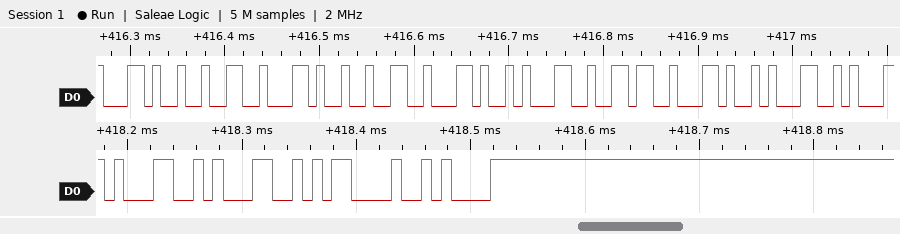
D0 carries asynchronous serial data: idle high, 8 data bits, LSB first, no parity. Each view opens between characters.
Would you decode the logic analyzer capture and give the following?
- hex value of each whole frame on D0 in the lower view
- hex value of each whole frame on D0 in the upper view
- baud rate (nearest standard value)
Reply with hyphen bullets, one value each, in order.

- 31, 31, 0D, 0A
- 2C, 32, 2C, 32, 2C, 31, 36, 2C, 31
- 115200 baud
